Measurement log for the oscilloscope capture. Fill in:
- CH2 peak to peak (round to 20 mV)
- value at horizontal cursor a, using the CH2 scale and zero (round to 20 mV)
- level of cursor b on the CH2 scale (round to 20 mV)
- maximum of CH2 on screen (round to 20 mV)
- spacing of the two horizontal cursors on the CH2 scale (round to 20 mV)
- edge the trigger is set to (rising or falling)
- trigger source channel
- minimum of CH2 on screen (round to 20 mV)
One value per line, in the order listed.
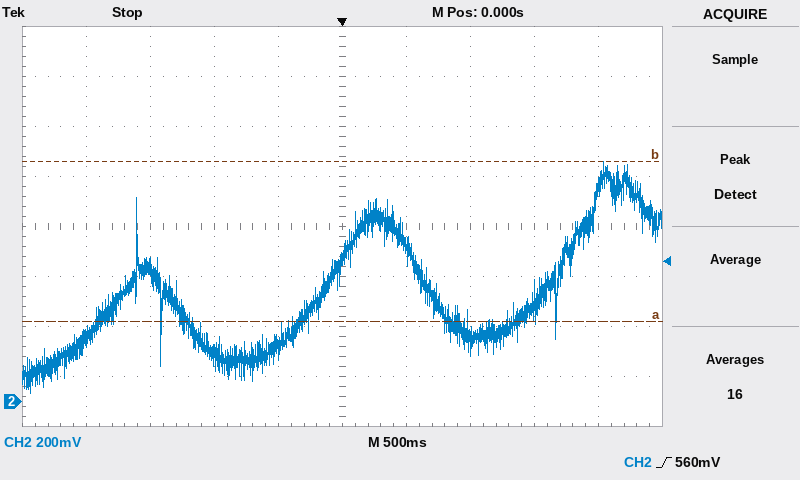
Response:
920 mV
320 mV
960 mV
960 mV
640 mV
rising
CH2
40 mV
